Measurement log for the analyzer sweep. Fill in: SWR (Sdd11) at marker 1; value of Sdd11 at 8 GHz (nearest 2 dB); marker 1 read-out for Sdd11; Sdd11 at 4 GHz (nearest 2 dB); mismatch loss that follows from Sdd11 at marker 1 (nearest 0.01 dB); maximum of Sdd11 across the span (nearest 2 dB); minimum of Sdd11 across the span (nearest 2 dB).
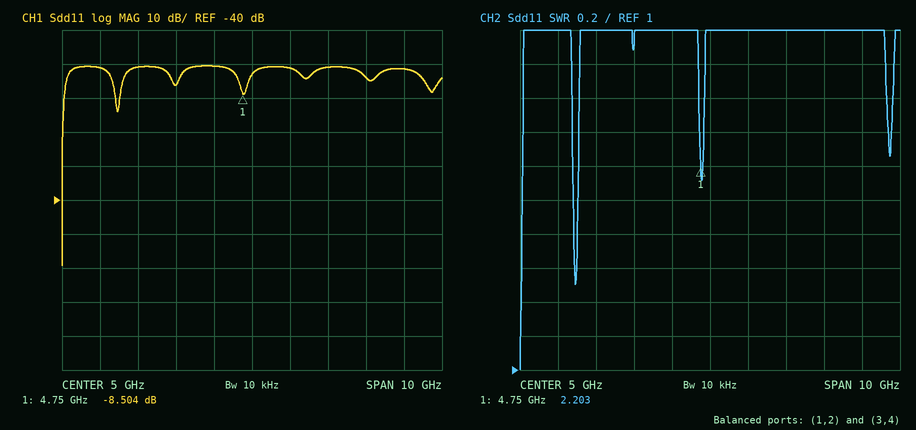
2.203
-4 dB
-8.504 dB
0 dB
0.66 dB
0 dB
-60 dB
